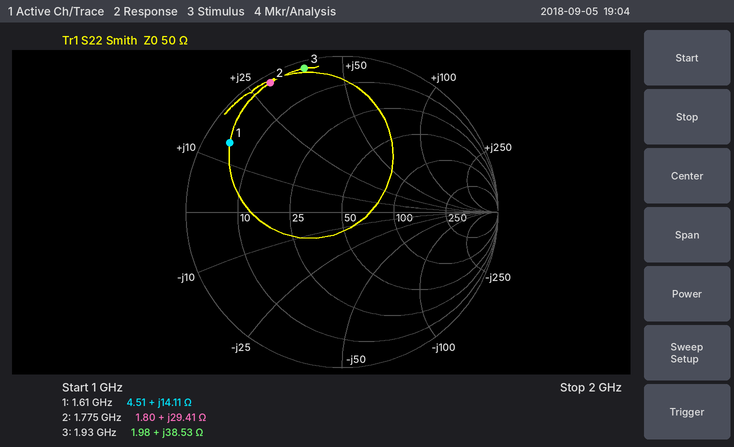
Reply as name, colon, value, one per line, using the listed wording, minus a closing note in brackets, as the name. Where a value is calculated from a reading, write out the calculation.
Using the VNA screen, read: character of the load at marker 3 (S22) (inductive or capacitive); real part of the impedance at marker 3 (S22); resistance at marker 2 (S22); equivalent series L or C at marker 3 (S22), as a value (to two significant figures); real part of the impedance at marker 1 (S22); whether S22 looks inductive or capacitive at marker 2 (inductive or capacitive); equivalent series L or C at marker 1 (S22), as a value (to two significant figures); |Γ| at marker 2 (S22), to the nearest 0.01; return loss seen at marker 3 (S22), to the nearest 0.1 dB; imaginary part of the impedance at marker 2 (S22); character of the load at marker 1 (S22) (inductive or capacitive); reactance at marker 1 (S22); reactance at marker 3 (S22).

character of the load at marker 3 (S22): inductive
real part of the impedance at marker 3: 1.98 Ω
resistance at marker 2: 1.80 Ω
equivalent series L or C at marker 3 (S22), as a value: L = 38.53 Ω/(2π × 1.93 GHz) ≈ 3.2 nH
real part of the impedance at marker 1: 4.51 Ω
whether S22 looks inductive or capacitive at marker 2: inductive
equivalent series L or C at marker 1 (S22), as a value: L = 14.11 Ω/(2π × 1.61 GHz) ≈ 1.4 nH
|Γ| at marker 2 (S22), to the nearest 0.01: 0.95
return loss seen at marker 3 (S22), to the nearest 0.1 dB: 0.4 dB
imaginary part of the impedance at marker 2: +29.41 Ω
character of the load at marker 1 (S22): inductive
reactance at marker 1: +14.11 Ω
reactance at marker 3: +38.53 Ω
